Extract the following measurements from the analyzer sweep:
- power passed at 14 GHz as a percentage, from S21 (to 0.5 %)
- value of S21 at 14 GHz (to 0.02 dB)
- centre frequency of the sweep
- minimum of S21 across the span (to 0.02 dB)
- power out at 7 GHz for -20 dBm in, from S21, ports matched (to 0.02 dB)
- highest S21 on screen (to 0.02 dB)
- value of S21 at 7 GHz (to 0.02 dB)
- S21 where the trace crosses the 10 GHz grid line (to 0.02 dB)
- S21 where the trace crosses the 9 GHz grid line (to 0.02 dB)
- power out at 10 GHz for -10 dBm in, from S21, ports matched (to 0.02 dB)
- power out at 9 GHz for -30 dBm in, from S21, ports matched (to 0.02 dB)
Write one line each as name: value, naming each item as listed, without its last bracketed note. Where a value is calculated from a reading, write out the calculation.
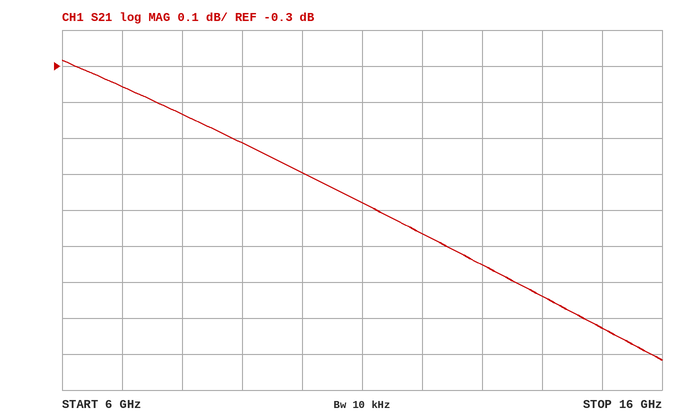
power passed at 14 GHz as a percentage, from S21: 10^(-0.94/10) ≈ 80.5 %
value of S21 at 14 GHz: -0.94 dB
centre frequency of the sweep: 11 GHz
minimum of S21 across the span: -1.12 dB
power out at 7 GHz for -20 dBm in, from S21, ports matched: -20 dBm + (-0.36 dB) = -20.36 dBm
highest S21 on screen: -0.28 dB
value of S21 at 7 GHz: -0.36 dB
S21 where the trace crosses the 10 GHz grid line: -0.60 dB
S21 where the trace crosses the 9 GHz grid line: -0.52 dB
power out at 10 GHz for -10 dBm in, from S21, ports matched: -10 dBm + (-0.60 dB) = -10.60 dBm
power out at 9 GHz for -30 dBm in, from S21, ports matched: -30 dBm + (-0.52 dB) = -30.52 dBm
